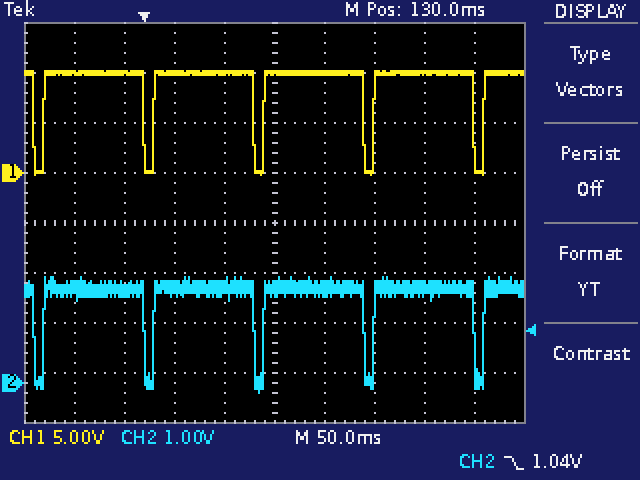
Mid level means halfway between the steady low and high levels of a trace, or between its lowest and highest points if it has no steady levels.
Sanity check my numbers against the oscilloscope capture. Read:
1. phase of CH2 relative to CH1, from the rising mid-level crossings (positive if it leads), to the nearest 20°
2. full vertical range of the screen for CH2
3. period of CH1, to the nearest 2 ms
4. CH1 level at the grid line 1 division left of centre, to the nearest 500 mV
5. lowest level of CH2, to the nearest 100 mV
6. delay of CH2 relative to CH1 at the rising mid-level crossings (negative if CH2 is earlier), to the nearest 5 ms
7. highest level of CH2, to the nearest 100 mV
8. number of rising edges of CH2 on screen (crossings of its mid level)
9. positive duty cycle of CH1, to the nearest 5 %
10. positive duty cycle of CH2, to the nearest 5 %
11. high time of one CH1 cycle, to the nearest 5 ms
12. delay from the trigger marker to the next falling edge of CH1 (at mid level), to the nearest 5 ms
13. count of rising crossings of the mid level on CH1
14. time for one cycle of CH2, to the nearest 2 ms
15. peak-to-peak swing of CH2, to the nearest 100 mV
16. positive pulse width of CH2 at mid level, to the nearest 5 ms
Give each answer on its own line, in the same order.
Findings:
0°
8 V
110 ms
10.0 V
-200 mV
0 ms
2.1 V
5
90 %
90 %
100 ms
110 ms
5
110 ms
2.3 V
100 ms
